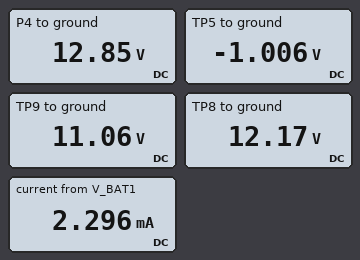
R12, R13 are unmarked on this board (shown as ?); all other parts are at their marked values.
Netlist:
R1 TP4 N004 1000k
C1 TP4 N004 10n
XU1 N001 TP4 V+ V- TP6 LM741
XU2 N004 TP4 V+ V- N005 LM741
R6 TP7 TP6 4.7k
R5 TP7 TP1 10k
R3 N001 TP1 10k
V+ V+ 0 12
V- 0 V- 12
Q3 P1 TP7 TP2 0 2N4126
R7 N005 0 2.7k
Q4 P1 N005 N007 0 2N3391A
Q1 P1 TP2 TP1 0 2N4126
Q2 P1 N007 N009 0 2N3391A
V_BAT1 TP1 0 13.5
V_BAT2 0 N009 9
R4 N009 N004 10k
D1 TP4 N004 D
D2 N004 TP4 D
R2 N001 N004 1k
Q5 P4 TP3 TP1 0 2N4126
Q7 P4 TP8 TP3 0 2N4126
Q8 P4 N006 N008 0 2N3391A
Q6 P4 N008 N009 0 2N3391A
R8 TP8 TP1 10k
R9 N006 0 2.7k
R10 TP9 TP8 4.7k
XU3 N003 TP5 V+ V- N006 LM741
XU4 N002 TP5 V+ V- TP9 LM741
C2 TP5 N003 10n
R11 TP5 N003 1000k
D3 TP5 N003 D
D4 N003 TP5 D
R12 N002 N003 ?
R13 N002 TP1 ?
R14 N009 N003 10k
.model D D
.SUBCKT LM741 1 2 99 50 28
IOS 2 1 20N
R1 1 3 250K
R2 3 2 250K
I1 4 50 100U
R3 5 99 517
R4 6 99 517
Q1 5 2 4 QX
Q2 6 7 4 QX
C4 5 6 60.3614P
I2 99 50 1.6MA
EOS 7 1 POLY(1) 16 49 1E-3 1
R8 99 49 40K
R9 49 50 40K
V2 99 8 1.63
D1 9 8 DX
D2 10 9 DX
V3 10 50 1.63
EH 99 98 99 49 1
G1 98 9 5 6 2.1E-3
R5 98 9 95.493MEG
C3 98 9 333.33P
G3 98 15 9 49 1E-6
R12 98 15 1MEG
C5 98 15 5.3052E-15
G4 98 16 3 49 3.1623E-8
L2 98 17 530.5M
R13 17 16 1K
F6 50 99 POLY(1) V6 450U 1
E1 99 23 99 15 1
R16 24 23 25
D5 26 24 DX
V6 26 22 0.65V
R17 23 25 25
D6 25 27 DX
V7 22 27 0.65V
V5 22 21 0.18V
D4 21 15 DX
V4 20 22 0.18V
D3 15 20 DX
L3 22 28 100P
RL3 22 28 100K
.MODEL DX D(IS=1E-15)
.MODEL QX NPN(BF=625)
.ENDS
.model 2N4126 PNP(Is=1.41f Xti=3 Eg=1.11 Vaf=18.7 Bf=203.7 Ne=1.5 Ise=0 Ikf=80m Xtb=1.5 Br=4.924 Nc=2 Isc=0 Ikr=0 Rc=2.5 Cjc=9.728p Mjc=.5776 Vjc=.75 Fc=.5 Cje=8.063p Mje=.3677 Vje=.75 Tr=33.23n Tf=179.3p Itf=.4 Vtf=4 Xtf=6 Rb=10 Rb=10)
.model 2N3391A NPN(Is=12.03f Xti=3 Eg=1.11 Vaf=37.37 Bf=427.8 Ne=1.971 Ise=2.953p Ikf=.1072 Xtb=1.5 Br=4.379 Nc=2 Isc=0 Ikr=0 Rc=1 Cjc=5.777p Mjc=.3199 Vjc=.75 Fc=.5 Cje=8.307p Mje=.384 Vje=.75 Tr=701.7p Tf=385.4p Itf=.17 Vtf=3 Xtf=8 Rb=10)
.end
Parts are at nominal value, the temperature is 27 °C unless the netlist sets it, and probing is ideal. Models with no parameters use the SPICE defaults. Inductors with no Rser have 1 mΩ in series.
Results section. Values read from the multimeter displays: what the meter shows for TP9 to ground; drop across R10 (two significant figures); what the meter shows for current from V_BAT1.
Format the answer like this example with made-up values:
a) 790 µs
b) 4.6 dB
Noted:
a) 11.06 V
b) 1.1 V
c) 2.296 mA
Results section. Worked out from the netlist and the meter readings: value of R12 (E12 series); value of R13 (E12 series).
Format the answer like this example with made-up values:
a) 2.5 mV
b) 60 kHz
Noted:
a) 1.8 kΩ
b) 18 kΩ
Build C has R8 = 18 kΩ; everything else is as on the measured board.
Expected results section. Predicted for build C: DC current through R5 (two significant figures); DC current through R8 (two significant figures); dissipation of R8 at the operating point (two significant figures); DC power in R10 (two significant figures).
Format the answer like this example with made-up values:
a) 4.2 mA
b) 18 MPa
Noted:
a) 130 µA
b) 75 µA
c) 100 µW
d) 250 µW
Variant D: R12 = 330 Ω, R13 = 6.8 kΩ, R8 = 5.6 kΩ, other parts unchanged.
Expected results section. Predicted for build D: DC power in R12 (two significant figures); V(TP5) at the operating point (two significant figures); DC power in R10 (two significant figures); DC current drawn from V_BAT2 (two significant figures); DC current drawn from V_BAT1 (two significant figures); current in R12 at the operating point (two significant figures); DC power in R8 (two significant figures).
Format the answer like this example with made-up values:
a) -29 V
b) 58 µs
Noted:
a) 570 µW
b) 4.3 V
c) 290 µW
d) 2.4 mA
e) 2.9 mA
f) 1.3 mA
g) 280 µW
